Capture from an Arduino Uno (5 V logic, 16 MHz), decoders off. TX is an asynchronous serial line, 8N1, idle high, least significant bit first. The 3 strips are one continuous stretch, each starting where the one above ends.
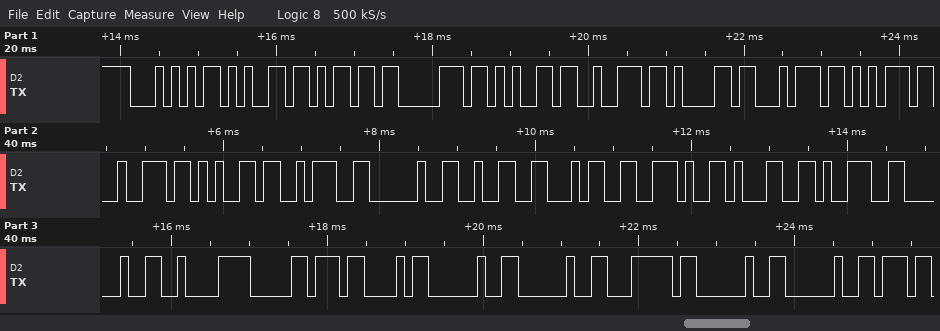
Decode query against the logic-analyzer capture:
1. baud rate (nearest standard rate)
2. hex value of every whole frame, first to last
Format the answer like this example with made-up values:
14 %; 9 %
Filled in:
9600 baud; 0x54 0x65 0x6D 0x70 0x65 0x72 0x61 0x74 0x75 0x72 0x65 0x3A 0x20 0x32 0x34 0x2E 0x31 0x39 0x20 0xC2 0xB0 0x43 0x20 0x20 0x7C 0x20 0x20
